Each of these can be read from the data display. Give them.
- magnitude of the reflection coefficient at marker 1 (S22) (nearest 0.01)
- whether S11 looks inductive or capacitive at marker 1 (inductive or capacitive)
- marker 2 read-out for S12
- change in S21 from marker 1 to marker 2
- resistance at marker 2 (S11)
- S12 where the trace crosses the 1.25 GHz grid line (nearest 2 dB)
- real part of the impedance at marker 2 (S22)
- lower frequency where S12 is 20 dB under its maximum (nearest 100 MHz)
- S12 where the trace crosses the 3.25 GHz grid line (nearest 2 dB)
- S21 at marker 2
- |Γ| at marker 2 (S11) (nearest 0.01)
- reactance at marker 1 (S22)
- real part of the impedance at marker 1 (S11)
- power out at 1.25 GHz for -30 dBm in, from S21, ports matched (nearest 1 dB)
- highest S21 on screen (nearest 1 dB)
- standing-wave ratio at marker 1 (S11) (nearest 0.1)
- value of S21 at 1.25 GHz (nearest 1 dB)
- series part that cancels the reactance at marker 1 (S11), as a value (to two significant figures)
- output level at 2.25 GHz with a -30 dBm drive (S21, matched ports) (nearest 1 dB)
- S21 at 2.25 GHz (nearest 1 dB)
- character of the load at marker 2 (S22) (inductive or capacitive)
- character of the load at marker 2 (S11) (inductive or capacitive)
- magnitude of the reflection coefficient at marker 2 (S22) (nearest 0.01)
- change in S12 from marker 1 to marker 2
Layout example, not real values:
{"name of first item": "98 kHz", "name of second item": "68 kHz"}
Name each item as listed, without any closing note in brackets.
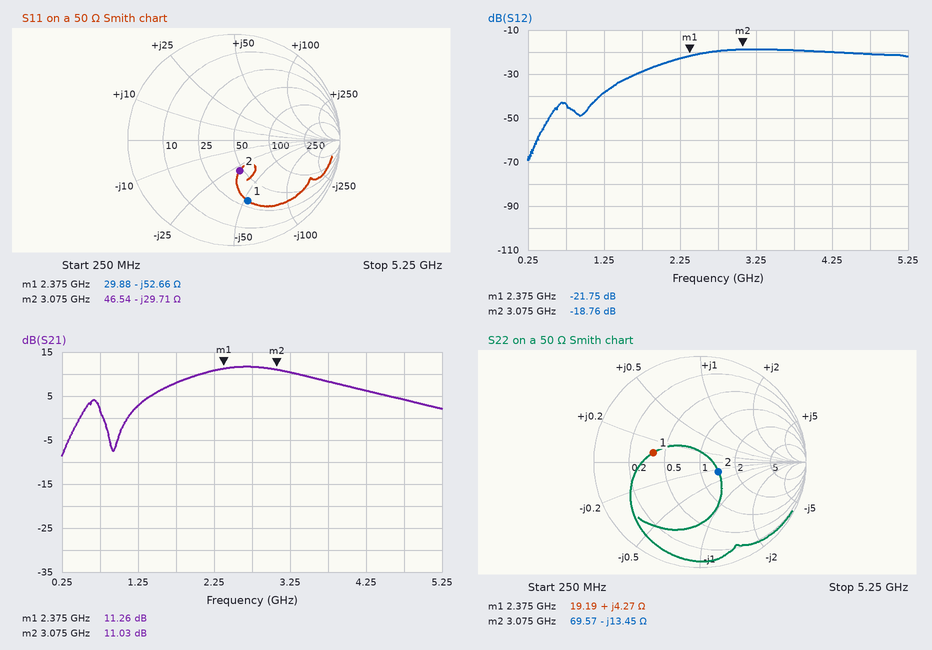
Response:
{"magnitude of the reflection coefficient at marker 1 (S22)": "0.45", "whether S11 looks inductive or capacitive at marker 1": "capacitive", "marker 2 read-out for S12": "-18.76 dB", "change in S21 from marker 1 to marker 2": "-0.23 dB", "resistance at marker 2": "46.54 Ω", "S12 where the trace crosses the 1.25 GHz grid line": "-38 dB", "real part of the impedance at marker 2": "69.57 Ω", "lower frequency where S12 is 20 dB under its maximum": "1.2 GHz", "S12 where the trace crosses the 3.25 GHz grid line": "-18 dB", "S21 at marker 2": "11.03 dB", "|Γ| at marker 2 (S11)": "0.30", "reactance at marker 1": "+4.27 Ω", "real part of the impedance at marker 1": "29.88 Ω", "power out at 1.25 GHz for -30 dBm in, from S21, ports matched": "-27 dBm", "highest S21 on screen": "12 dB", "standing-wave ratio at marker 1 (S11)": "3.9", "value of S21 at 1.25 GHz": "3 dB", "series part that cancels the reactance at marker 1 (S11), as a value": "3.5 nH", "output level at 2.25 GHz with a -30 dBm drive (S21, matched ports)": "-19 dBm", "S21 at 2.25 GHz": "11 dB", "character of the load at marker 2 (S22)": "capacitive", "character of the load at marker 2 (S11)": "capacitive", "magnitude of the reflection coefficient at marker 2 (S22)": "0.20", "change in S12 from marker 1 to marker 2": "2.99 dB"}
